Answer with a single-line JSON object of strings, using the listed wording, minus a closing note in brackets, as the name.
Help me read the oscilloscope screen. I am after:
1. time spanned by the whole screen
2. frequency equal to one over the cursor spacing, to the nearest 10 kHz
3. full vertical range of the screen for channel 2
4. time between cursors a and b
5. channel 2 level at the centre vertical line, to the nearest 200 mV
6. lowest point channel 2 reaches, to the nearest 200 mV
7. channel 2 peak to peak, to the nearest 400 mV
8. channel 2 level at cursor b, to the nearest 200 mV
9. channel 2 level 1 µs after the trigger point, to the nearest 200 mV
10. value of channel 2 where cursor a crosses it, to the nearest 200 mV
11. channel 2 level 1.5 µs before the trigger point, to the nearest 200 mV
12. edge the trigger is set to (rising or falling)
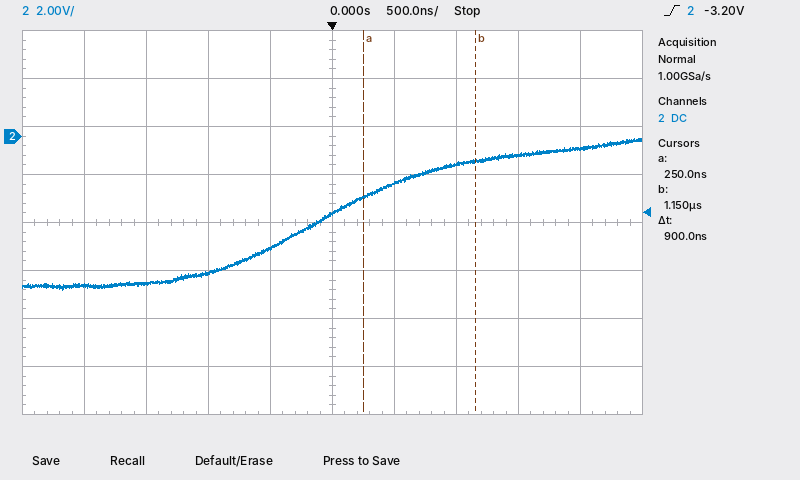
{"time spanned by the whole screen": "5 µs", "frequency equal to one over the cursor spacing, to the nearest 10 kHz": "1.11 MHz", "full vertical range of the screen for channel 2": "16 V", "time between cursors a and b": "900 ns", "channel 2 level at the centre vertical line, to the nearest 200 mV": "-3.2 V", "lowest point channel 2 reaches, to the nearest 200 mV": "-6.4 V", "channel 2 peak to peak, to the nearest 400 mV": "6.4 V", "channel 2 level at cursor b, to the nearest 200 mV": "-1.0 V", "channel 2 level 1 µs after the trigger point, to the nearest 200 mV": "-1.2 V", "value of channel 2 where cursor a crosses it, to the nearest 200 mV": "-2.6 V", "channel 2 level 1.5 µs before the trigger point, to the nearest 200 mV": "-6.2 V", "edge the trigger is set to": "rising"}
